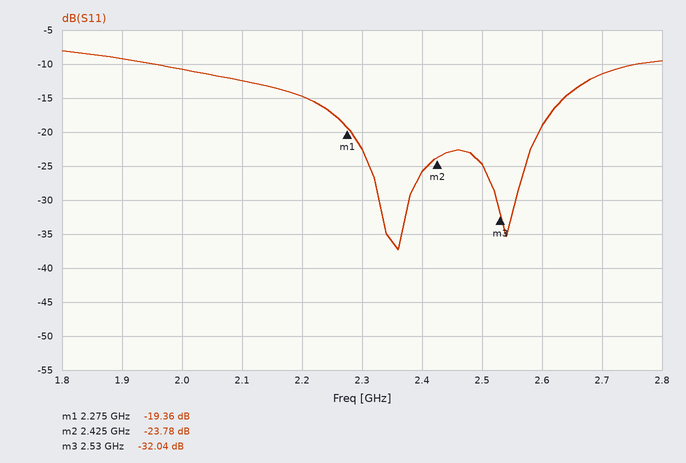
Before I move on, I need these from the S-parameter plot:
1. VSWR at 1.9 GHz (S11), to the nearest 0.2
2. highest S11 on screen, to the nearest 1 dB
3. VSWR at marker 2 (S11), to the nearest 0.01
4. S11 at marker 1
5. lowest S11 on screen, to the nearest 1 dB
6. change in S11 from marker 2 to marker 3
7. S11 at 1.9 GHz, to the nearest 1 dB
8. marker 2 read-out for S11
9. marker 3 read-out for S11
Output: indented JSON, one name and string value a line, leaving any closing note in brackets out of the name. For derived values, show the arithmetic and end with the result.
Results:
{
  "VSWR at 1.9 GHz (S11), to the nearest 0.2": "|Γ| = 10^(-9/20) = 0.3548; VSWR = (1 + 0.3548)/(1 − 0.3548) ≈ 2.10, so 2.0 to the nearest 0.2",
  "highest S11 on screen, to the nearest 1 dB": "-8 dB",
  "VSWR at marker 2 (S11), to the nearest 0.01": "(1 + 0.0647)/(1 − 0.0647) ≈ 1.14",
  "S11 at marker 1": "-19.36 dB",
  "lowest S11 on screen, to the nearest 1 dB": "-37 dB",
  "change in S11 from marker 2 to marker 3": "-32.04 − (-23.78) = -8.26 dB",
  "S11 at 1.9 GHz, to the nearest 1 dB": "-9 dB",
  "marker 2 read-out for S11": "-23.78 dB",
  "marker 3 read-out for S11": "-32.04 dB"
}
